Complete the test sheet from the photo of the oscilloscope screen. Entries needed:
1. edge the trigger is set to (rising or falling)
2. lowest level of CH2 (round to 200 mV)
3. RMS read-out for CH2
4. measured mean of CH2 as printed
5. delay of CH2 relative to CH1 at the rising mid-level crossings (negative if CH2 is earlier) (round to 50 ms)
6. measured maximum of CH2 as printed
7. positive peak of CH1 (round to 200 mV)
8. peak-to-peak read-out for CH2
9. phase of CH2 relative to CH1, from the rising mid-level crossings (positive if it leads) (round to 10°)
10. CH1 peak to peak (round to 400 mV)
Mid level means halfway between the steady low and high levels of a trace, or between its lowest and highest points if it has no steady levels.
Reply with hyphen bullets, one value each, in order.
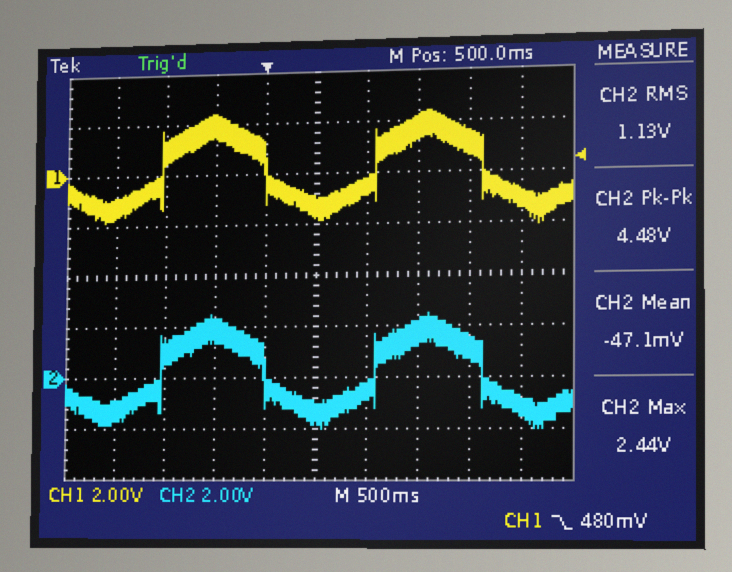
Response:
- falling
- -2.0 V
- 1.13 V
- -47.1 mV
- 0 ms
- 2.44 V
- 2.4 V
- 4.48 V
- 0°
- 4.4 V
